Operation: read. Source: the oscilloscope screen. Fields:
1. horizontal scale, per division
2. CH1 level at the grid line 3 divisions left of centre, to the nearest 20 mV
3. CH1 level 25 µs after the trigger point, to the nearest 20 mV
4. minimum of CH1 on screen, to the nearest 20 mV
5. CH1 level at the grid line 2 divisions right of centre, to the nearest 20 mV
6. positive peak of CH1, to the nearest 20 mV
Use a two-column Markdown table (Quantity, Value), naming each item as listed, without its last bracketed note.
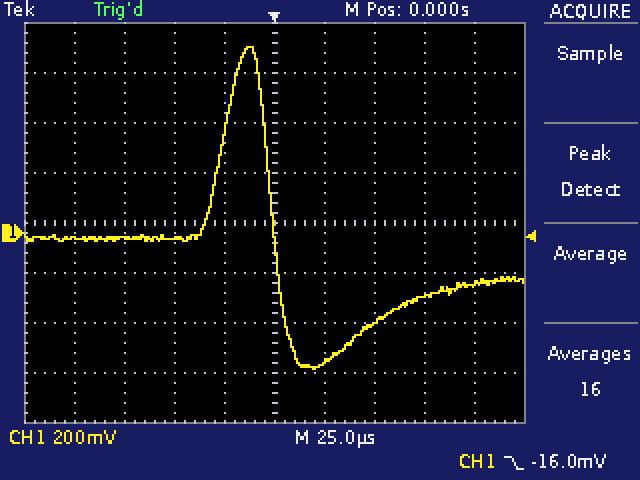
| Quantity | Value |
|---|---|
| horizontal scale, per division | 25 µs |
| CH1 level at the grid line 3 divisions left of centre, to the nearest 20 mV | -20 mV |
| CH1 level 25 µs after the trigger point, to the nearest 20 mV | -520 mV |
| minimum of CH1 on screen, to the nearest 20 mV | -540 mV |
| CH1 level at the grid line 2 divisions right of centre, to the nearest 20 mV | -360 mV |
| positive peak of CH1, to the nearest 20 mV | 740 mV |
